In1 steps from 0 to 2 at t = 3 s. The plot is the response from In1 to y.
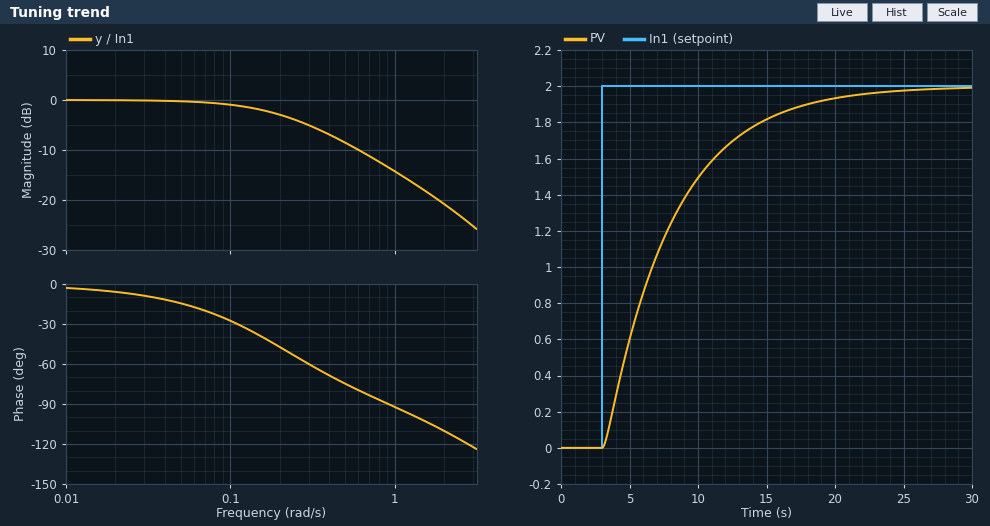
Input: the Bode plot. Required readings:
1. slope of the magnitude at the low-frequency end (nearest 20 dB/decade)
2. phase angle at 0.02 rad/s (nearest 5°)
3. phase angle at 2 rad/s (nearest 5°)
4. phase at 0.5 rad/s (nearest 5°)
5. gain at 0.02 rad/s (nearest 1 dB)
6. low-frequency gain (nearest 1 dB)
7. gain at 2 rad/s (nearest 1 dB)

0 dB/decade
-5°
-110°
-75°
0 dB
0 dB
-21 dB
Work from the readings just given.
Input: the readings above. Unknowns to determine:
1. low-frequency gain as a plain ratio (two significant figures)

1.0
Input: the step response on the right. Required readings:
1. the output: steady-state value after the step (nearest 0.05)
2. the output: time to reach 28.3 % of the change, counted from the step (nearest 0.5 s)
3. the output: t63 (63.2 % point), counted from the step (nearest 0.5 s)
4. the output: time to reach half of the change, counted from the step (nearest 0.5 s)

2.00
2.0 s
5.0 s
3.5 s
